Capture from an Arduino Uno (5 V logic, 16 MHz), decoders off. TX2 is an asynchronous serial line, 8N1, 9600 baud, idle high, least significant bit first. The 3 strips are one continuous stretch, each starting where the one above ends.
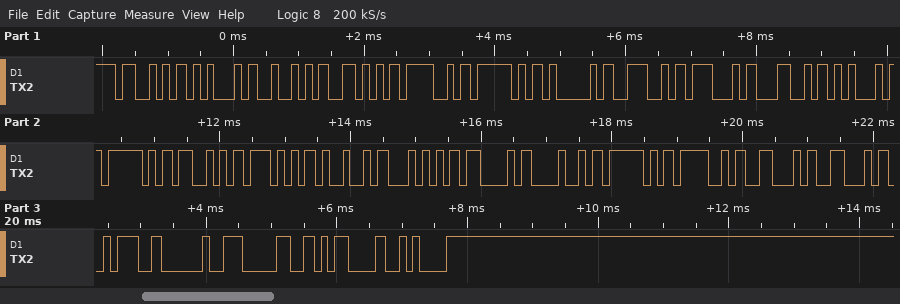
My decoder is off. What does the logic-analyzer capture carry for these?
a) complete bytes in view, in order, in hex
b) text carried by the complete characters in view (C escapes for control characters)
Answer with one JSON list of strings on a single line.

["53 45 52 56 4F 5F 41 4E 47 4C 45 5F 53 57 49 54 43 48 5F 4F 46 46 3A 20 30 0D 0A", "\"SERVO_ANGLE_SWITCH_OFF: 0\\r\\n\""]
